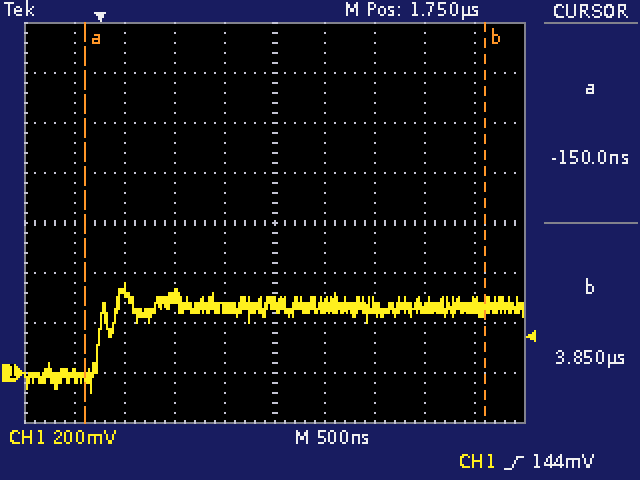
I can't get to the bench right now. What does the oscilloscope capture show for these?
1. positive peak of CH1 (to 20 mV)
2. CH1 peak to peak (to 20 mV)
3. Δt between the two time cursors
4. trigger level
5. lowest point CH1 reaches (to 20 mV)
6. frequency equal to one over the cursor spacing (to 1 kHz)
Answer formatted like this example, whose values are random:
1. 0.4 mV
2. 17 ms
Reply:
1. 360 mV
2. 440 mV
3. 4.00 µs
4. 144 mV
5. -80 mV
6. 250 kHz
